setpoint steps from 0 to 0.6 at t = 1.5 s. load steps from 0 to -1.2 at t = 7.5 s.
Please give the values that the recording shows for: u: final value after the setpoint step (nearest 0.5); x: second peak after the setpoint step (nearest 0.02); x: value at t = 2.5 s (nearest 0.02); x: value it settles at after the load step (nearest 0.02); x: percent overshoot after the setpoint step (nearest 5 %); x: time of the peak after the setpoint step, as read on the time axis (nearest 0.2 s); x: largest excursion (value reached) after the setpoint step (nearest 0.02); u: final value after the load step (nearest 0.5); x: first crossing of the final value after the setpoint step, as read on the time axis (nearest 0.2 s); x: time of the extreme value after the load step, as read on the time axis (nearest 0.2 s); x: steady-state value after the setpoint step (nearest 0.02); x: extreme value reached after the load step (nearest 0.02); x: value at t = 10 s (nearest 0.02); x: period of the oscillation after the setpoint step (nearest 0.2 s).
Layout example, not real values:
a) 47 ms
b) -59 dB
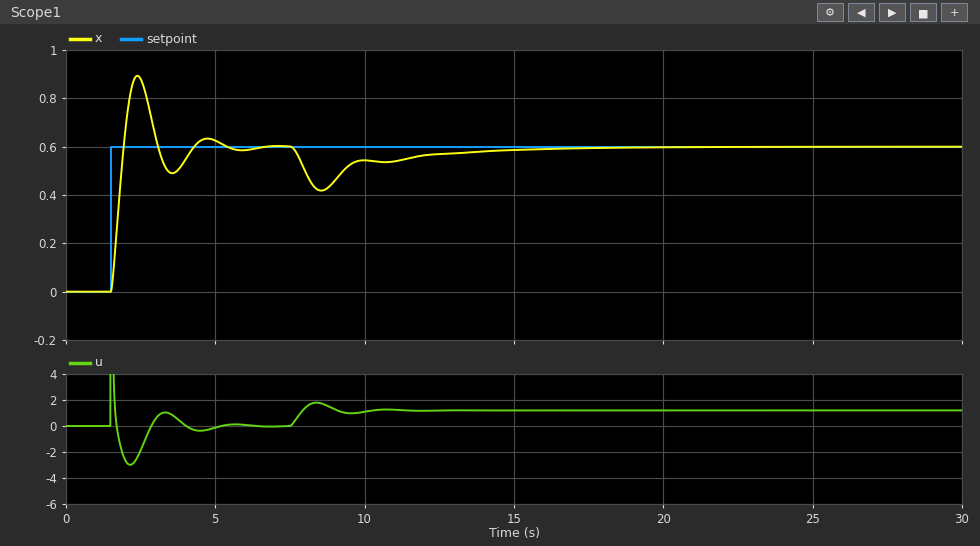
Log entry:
a) 0.0
b) 0.64
c) 0.88
d) 0.60
e) 50 %
f) 2.4 s
g) 0.90
h) 1.0
i) 2.0 s
j) 8.6 s
k) 0.60
l) 0.42
m) 0.54
n) 2.4 s
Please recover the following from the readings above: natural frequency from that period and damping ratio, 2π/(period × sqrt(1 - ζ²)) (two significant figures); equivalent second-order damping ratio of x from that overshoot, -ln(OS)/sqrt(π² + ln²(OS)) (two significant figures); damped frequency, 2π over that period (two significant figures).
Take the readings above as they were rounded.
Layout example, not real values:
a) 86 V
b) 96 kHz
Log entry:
a) 2.7 rad/s
b) 0.22
c) 2.6 rad/s
